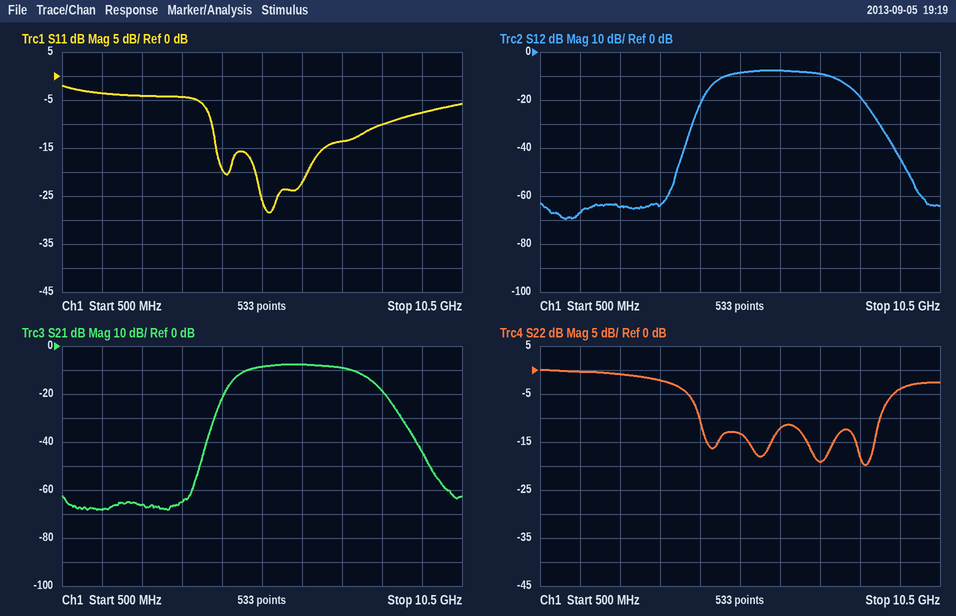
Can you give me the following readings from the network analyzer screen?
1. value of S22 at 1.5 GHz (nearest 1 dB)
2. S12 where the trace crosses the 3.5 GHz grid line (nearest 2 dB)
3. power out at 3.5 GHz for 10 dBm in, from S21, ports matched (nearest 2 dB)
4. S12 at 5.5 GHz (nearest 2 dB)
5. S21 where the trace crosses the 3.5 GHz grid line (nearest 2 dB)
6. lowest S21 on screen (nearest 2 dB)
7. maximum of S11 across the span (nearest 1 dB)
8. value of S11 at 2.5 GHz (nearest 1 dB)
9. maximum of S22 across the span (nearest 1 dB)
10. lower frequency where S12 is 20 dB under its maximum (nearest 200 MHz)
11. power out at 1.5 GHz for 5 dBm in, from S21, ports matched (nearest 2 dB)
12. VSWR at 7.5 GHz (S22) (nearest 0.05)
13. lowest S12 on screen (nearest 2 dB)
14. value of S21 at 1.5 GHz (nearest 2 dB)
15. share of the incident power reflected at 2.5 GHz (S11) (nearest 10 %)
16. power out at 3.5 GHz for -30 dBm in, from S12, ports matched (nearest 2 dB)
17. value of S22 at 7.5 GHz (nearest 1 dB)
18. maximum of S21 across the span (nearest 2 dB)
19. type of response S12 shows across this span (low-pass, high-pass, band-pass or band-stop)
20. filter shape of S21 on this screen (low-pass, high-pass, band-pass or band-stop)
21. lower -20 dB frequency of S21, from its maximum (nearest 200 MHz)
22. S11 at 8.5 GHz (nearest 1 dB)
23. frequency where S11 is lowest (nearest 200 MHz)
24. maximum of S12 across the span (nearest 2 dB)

0 dB
-64 dB
-54 dBm
-8 dB
-64 dB
-68 dB
-2 dB
-4 dB
0 dB
4.4 GHz
-64 dBm
1.25
-70 dB
-68 dB
40 %
-94 dBm
-19 dB
-8 dB
band-pass
band-pass
4.4 GHz
-10 dB
5.6 GHz
-8 dB
